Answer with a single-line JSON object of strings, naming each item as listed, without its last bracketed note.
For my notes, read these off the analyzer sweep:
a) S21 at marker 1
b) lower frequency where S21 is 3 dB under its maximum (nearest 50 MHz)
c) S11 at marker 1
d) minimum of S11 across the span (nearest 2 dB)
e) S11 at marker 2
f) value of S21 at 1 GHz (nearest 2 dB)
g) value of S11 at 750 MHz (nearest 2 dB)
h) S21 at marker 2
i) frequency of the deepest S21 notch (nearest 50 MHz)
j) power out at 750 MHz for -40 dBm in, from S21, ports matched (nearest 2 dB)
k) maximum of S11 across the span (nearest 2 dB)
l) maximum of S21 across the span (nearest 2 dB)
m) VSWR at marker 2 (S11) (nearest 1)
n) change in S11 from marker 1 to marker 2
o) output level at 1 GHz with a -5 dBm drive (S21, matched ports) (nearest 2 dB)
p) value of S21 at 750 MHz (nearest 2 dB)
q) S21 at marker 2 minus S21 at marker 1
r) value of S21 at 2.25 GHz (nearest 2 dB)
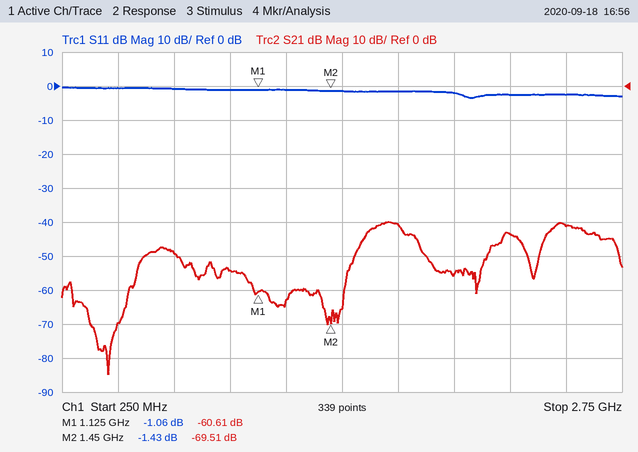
{"S21 at marker 1": "-60.61 dB", "lower frequency where S21 is 3 dB under its maximum": "1.60 GHz", "S11 at marker 1": "-1.06 dB", "minimum of S11 across the span": "-4 dB", "S11 at marker 2": "-1.43 dB", "value of S21 at 1 GHz": "-54 dB", "value of S11 at 750 MHz": "0 dB", "S21 at marker 2": "-69.51 dB", "frequency of the deepest S21 notch": "450 MHz", "power out at 750 MHz for -40 dBm in, from S21, ports matched": "-90 dBm", "maximum of S11 across the span": "0 dB", "maximum of S21 across the span": "-40 dB", "VSWR at marker 2 (S11)": "12", "change in S11 from marker 1 to marker 2": "-0.37 dB", "output level at 1 GHz with a -5 dBm drive (S21, matched ports)": "-60 dBm", "value of S21 at 750 MHz": "-50 dB", "S21 at marker 2 minus S21 at marker 1": "-8.90 dB", "value of S21 at 2.25 GHz": "-44 dB"}
